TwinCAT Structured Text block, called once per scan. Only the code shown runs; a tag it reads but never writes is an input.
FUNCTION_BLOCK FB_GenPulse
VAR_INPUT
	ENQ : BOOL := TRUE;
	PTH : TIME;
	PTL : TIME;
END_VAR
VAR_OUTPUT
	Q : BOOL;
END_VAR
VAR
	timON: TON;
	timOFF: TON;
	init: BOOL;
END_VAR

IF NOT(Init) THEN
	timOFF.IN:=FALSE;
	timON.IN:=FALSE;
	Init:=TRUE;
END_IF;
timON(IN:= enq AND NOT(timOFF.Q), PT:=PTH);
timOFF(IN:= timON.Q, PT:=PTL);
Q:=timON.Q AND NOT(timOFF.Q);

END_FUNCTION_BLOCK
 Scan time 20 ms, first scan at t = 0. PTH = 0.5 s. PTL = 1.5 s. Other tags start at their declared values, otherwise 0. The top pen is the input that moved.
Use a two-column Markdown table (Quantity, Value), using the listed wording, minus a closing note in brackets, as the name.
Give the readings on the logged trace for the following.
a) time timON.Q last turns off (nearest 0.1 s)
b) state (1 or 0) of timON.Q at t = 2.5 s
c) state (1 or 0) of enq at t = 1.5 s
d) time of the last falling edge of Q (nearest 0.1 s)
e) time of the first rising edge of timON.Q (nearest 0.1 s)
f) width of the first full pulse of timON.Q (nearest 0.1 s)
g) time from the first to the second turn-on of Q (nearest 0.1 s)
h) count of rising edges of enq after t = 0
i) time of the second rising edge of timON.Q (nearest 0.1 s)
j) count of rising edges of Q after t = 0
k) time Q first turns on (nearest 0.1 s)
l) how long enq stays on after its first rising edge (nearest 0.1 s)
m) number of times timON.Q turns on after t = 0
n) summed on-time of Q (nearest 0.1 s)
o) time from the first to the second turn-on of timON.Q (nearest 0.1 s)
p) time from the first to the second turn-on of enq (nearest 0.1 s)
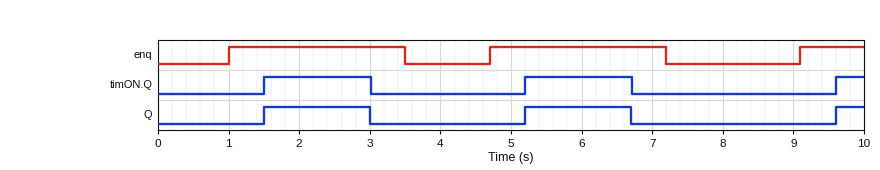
| Quantity | Value |
|---|---|
| time timON.Q last turns off | 6.7 s |
| state (1 or 0) of timON.Q at t = 2.5 s | 1 |
| state (1 or 0) of enq at t = 1.5 s | 1 |
| time of the last falling edge of Q | 6.7 s |
| time of the first rising edge of timON.Q | 1.5 s |
| width of the first full pulse of timON.Q | 1.5 s |
| time from the first to the second turn-on of Q | 3.7 s |
| count of rising edges of enq after t = 0 | 3 |
| time of the second rising edge of timON.Q | 5.2 s |
| count of rising edges of Q after t = 0 | 3 |
| time Q first turns on | 1.5 s |
| how long enq stays on after its first rising edge | 2.5 s |
| number of times timON.Q turns on after t = 0 | 3 |
| summed on-time of Q | 3.4 s |
| time from the first to the second turn-on of timON.Q | 3.7 s |
| time from the first to the second turn-on of enq | 3.7 s |
